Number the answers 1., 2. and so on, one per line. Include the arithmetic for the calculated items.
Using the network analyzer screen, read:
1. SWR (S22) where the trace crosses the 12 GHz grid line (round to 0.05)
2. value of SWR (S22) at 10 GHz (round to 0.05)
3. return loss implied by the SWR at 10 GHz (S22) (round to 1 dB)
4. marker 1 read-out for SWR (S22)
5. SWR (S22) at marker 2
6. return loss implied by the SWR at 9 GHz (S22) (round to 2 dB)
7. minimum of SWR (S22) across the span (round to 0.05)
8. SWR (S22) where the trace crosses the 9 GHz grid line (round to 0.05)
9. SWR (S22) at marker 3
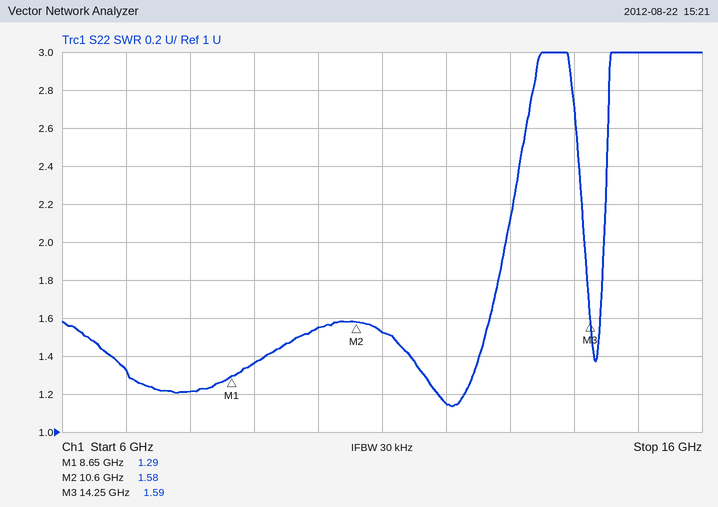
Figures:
1. 1.15
2. 1.55
3. −20 log10((1.55 − 1)/(1.55 + 1)) ≈ 13 dB
4. 1.29
5. 1.58
6. −20 log10((1.35 − 1)/(1.35 + 1)) ≈ 16 dB
7. 1.15
8. 1.35
9. 1.59
